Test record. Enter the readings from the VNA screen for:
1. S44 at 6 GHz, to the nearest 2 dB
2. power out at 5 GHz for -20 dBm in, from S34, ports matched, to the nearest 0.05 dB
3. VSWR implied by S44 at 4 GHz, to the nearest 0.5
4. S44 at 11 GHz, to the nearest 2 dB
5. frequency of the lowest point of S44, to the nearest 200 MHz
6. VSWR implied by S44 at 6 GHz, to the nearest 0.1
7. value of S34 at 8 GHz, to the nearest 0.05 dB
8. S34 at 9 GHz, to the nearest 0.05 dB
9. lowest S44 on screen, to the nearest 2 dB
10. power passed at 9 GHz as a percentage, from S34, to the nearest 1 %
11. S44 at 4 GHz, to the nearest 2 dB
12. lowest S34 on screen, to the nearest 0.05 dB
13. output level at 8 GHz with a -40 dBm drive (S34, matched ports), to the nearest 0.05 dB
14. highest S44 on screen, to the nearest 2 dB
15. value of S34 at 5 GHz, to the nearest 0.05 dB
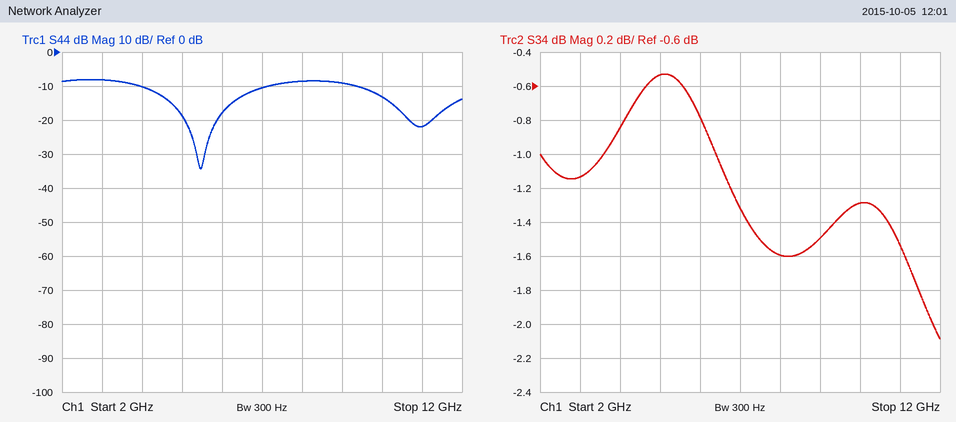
-18 dB
-20.55 dBm
2.0
-22 dB
5.4 GHz
1.3
-1.60 dB
-1.50 dB
-34 dB
71 %
-10 dB
-2.10 dB
-41.60 dBm
-8 dB
-0.55 dB
